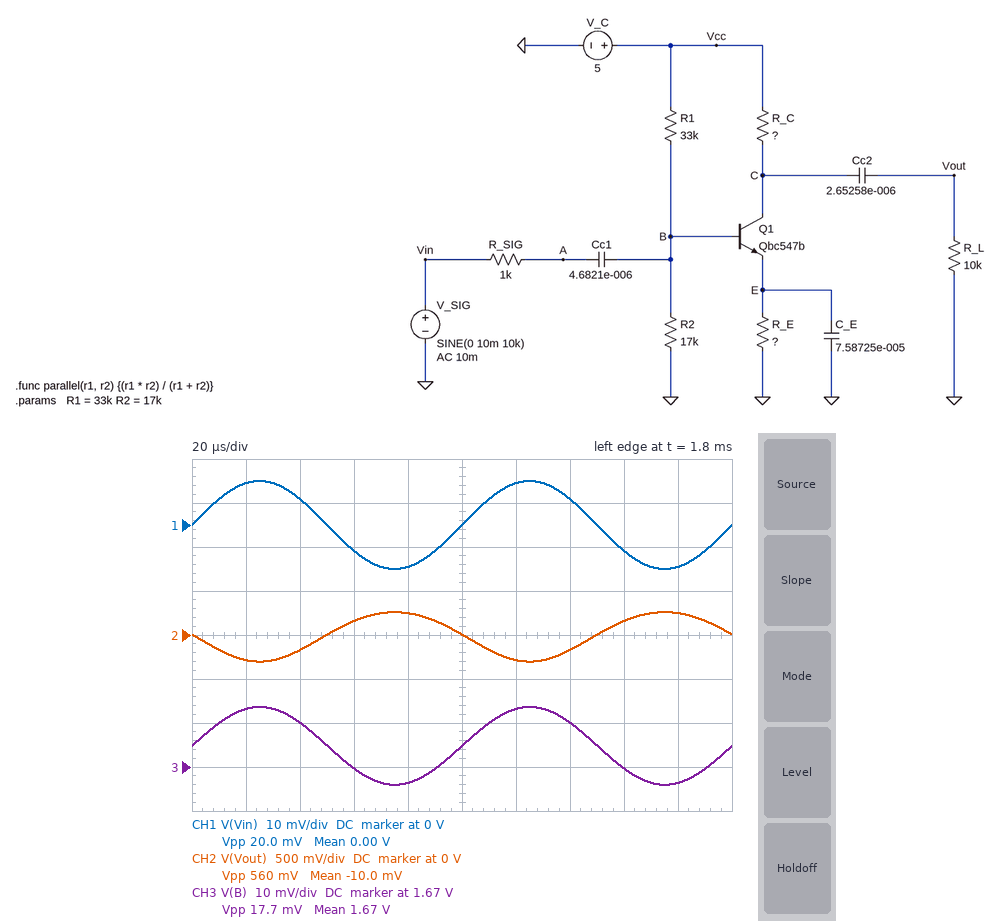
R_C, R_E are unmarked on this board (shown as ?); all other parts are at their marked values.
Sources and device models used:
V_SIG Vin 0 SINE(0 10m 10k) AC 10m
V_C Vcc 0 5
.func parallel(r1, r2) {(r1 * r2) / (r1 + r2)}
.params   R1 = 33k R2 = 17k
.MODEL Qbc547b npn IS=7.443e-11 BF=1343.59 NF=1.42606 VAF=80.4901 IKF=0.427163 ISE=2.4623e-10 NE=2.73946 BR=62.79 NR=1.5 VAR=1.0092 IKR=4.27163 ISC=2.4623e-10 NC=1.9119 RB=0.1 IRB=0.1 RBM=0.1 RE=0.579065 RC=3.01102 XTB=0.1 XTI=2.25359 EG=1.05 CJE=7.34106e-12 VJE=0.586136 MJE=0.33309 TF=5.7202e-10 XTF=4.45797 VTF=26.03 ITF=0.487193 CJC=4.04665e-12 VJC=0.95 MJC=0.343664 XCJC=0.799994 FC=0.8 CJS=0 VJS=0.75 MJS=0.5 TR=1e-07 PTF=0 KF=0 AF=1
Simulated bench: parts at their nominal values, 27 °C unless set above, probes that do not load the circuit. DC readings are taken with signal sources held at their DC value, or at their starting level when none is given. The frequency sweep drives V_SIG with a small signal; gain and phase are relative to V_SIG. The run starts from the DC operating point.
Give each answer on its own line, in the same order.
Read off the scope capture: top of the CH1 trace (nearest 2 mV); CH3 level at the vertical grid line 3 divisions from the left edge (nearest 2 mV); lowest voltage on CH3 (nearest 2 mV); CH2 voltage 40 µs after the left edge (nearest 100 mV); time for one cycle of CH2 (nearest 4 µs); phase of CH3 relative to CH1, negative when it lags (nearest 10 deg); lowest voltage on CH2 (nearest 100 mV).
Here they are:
10 mV
1.670 V
1.666 V
-200 mV
100 µs
0 deg
-300 mV
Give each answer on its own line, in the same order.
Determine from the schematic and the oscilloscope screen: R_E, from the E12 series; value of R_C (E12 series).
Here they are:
2.2 kΩ
3.9 kΩ
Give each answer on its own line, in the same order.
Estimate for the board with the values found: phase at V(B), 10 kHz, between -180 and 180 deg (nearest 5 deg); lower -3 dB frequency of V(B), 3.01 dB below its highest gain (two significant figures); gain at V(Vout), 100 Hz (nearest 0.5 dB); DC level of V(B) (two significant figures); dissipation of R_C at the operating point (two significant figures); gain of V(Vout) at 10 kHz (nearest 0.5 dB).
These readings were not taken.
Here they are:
0 deg
2.8 Hz
28.5 dB
1.7 V
900 µW
29.0 dB
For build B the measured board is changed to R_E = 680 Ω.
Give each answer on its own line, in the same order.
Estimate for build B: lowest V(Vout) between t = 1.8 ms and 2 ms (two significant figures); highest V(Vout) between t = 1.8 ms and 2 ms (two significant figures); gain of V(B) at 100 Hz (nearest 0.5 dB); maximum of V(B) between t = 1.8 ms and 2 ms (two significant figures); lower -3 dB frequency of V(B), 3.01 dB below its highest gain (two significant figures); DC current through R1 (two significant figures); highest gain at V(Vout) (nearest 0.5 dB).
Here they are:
-14 mV
21 mV
-17.5 dB
1.4 V
8.0 Hz
110 µA
4.5 dB
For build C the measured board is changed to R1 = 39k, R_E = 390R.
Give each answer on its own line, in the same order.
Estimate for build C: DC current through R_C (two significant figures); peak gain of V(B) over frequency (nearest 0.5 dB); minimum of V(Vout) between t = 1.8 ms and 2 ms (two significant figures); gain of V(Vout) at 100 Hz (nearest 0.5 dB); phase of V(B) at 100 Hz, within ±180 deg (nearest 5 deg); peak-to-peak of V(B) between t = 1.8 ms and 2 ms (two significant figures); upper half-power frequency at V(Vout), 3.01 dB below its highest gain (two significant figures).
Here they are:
1.1 mA
-18.0 dB
-11 mV
1.5 dB
5 deg
2.5 mV
220 kHz
